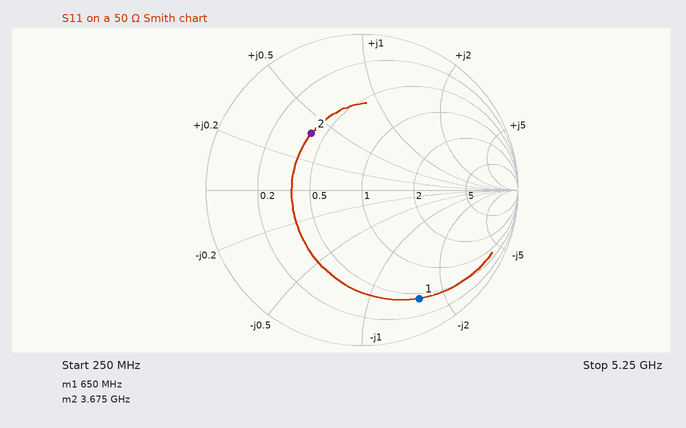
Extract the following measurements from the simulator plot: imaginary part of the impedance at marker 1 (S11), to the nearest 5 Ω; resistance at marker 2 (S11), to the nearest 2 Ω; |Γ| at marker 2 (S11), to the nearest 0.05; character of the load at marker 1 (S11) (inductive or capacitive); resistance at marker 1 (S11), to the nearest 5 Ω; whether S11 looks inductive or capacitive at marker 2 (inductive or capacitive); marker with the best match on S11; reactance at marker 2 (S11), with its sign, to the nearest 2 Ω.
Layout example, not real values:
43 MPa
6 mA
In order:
-80 Ω
20 Ω
0.50
capacitive
20 Ω
inductive
marker 2
+20 Ω
